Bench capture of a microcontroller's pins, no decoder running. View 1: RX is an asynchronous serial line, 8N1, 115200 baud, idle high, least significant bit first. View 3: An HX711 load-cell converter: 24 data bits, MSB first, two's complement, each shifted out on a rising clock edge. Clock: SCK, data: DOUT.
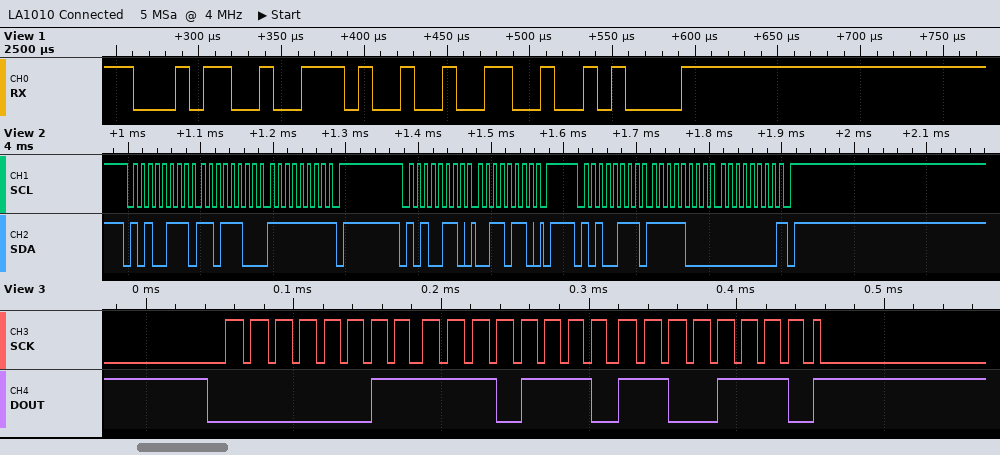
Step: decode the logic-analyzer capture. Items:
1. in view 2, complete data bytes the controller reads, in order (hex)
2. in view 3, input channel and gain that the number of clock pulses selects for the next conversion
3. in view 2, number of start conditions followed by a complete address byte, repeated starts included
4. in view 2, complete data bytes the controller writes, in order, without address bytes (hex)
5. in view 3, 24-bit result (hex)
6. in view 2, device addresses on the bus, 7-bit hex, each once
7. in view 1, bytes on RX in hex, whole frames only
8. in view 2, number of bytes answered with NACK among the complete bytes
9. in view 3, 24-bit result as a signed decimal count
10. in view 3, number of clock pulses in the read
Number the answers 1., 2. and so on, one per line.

1. DC FF F8 00
2. channel A, gain 128
3. 3
4. 36
5. 0x03EECE
6. 0x53
7. 0x34 0x2E 0x32 0x0A
8. 2
9. 257742
10. 25
